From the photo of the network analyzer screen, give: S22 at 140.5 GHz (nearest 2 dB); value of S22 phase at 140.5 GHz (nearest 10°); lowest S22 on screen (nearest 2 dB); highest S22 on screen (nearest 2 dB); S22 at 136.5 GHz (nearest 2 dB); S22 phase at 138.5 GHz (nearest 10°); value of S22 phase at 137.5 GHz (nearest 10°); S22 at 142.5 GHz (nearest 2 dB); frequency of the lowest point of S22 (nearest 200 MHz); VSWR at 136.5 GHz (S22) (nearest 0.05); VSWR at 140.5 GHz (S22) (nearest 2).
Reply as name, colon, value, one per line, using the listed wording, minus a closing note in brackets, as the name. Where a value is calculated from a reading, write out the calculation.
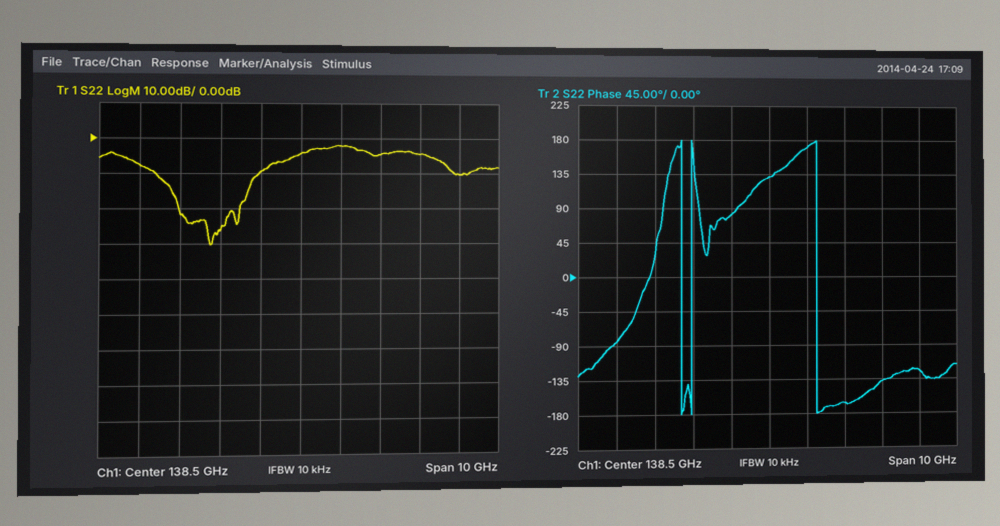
S22 at 140.5 GHz: -4 dB
value of S22 phase at 140.5 GHz: -170°
lowest S22 on screen: -30 dB
highest S22 on screen: -2 dB
S22 at 136.5 GHz: -26 dB
S22 phase at 138.5 GHz: 130°
value of S22 phase at 137.5 GHz: 80°
S22 at 142.5 GHz: -10 dB
frequency of the lowest point of S22: 136.2 GHz
VSWR at 136.5 GHz (S22): |Γ| = 10^(-26/20) = 0.0501; VSWR = (1 + 0.0501)/(1 − 0.0501) ≈ 1.11, so 1.10 to the nearest 0.05
VSWR at 140.5 GHz (S22): |Γ| = 10^(-4/20) = 0.6310; VSWR = (1 + 0.6310)/(1 − 0.6310) ≈ 4
